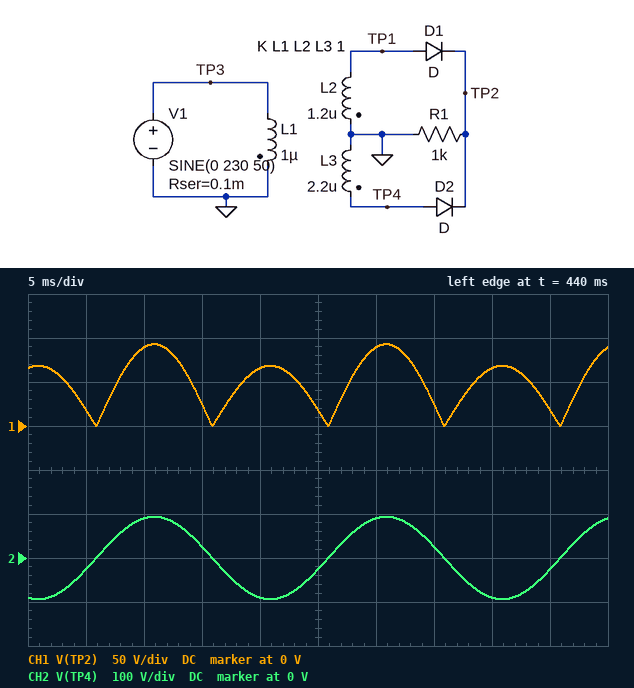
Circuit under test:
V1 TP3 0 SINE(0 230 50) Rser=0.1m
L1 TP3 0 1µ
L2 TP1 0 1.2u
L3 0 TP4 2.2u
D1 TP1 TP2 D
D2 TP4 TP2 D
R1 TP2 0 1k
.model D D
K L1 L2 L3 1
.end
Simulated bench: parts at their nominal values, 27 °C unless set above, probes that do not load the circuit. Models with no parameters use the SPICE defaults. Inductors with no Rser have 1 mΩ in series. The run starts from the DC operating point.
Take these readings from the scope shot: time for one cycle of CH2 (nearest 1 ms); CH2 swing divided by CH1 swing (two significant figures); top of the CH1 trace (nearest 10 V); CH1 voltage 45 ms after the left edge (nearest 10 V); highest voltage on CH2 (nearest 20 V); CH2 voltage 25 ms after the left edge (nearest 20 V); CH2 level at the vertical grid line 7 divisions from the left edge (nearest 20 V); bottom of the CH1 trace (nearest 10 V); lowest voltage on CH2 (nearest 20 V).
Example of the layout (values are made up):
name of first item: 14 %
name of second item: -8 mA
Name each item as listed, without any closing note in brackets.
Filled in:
time for one cycle of CH2: 20 ms
CH2 swing divided by CH1 swing: 2.0
top of the CH1 trace: 90 V
CH1 voltage 45 ms after the left edge: 20 V
highest voltage on CH2: 100 V
CH2 voltage 25 ms after the left edge: -20 V
CH2 level at the vertical grid line 7 divisions from the left edge: 20 V
bottom of the CH1 trace: 0 V
lowest voltage on CH2: -100 V
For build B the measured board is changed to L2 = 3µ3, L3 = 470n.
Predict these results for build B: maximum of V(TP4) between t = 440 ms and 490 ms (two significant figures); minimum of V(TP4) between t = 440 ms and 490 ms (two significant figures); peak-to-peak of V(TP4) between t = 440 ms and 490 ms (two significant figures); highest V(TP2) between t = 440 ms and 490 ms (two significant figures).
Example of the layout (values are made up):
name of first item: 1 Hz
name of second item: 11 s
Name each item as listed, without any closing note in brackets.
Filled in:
maximum of V(TP4) between t = 440 ms and 490 ms: 43 V
minimum of V(TP4) between t = 440 ms and 490 ms: -43 V
peak-to-peak of V(TP4) between t = 440 ms and 490 ms: 87 V
highest V(TP2) between t = 440 ms and 490 ms: 110 V
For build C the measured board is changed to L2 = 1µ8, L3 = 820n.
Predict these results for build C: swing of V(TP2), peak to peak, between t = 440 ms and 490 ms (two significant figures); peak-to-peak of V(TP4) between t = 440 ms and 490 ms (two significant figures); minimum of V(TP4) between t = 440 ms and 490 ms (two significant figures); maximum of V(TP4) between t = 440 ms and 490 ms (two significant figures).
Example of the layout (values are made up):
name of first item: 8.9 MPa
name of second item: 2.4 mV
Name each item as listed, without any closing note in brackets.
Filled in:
swing of V(TP2), peak to peak, between t = 440 ms and 490 ms: 84 V
peak-to-peak of V(TP4) between t = 440 ms and 490 ms: 110 V
minimum of V(TP4) between t = 440 ms and 490 ms: -57 V
maximum of V(TP4) between t = 440 ms and 490 ms: 57 V
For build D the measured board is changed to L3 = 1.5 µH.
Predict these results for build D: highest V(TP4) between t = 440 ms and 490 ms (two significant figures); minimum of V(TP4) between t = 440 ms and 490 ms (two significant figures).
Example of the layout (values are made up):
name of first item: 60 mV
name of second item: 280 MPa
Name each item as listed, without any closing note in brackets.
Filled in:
highest V(TP4) between t = 440 ms and 490 ms: 77 V
minimum of V(TP4) between t = 440 ms and 490 ms: -77 V
